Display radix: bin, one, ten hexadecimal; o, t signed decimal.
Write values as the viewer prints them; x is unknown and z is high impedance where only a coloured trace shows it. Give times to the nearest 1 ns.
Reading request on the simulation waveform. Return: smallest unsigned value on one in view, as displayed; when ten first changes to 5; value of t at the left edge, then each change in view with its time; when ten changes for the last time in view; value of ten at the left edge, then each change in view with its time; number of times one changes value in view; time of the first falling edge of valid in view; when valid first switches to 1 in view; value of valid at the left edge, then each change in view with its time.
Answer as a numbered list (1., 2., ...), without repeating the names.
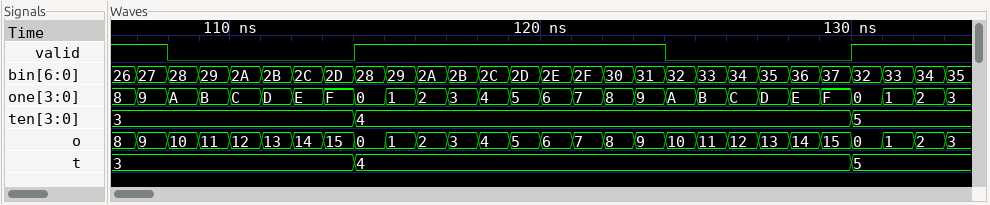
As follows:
1. 0
2. 130 ns
3. 3, 4 at 114 ns, 5 at 130 ns
4. 130 ns
5. 3, 4 at 114 ns, 5 at 130 ns
6. 27
7. 108 ns
8. 114 ns
9. 1, 0 at 108 ns, 1 at 114 ns, 0 at 124 ns, 1 at 130 ns
